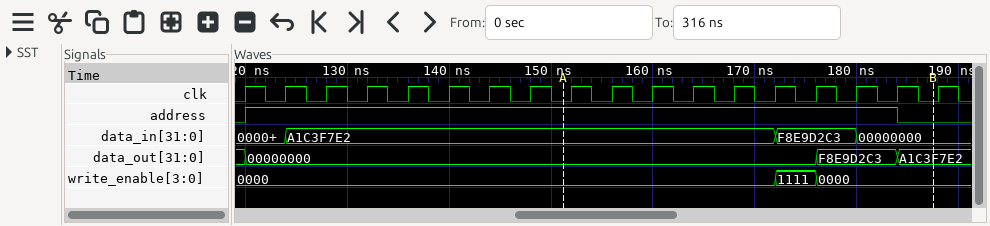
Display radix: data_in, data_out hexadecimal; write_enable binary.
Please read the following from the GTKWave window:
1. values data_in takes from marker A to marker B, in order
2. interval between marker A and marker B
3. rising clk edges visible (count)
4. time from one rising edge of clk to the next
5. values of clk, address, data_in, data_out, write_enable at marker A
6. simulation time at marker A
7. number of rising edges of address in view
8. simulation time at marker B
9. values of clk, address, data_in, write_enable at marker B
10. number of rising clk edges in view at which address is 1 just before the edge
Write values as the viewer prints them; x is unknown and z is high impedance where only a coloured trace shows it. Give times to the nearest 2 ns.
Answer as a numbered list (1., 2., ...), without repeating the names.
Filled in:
1. A1C3F7E2, F8E9D2C3, 00000000
2. 36 ns
3. 18
4. 4 ns
5. clk=0, address=1, data_in=A1C3F7E2, data_out=00000000, write_enable=0000
6. 152 ns
7. 1
8. 188 ns
9. clk=0, address=0, data_in=00000000, write_enable=0000
10. 16
